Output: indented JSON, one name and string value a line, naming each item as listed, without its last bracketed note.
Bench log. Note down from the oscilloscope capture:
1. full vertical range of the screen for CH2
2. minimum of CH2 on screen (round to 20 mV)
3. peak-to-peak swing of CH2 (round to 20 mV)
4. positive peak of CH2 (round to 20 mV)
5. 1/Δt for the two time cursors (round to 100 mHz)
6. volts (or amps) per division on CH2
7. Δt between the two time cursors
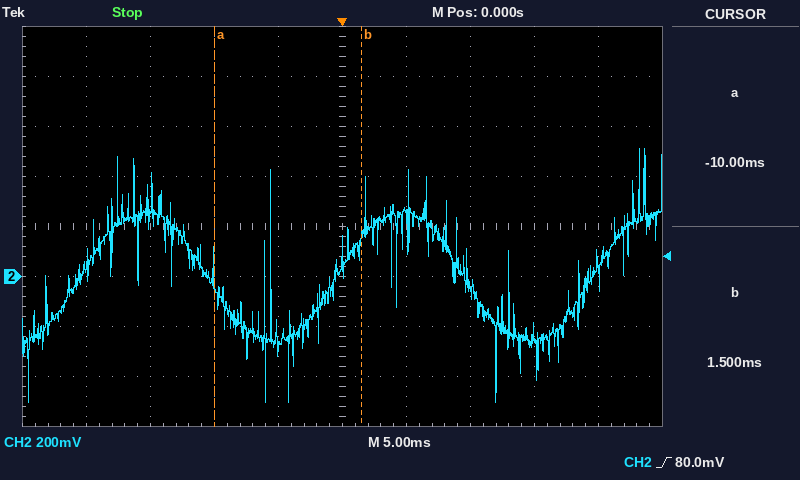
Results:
{
  "full vertical range of the screen for CH2": "1.6 V",
  "minimum of CH2 on screen": "-500 mV",
  "peak-to-peak swing of CH2": "1.02 V",
  "positive peak of CH2": "520 mV",
  "1/Δt for the two time cursors": "87.0 Hz",
  "volts (or amps) per division on CH2": "200 mV",
  "Δt between the two time cursors": "11.5 ms"
}
